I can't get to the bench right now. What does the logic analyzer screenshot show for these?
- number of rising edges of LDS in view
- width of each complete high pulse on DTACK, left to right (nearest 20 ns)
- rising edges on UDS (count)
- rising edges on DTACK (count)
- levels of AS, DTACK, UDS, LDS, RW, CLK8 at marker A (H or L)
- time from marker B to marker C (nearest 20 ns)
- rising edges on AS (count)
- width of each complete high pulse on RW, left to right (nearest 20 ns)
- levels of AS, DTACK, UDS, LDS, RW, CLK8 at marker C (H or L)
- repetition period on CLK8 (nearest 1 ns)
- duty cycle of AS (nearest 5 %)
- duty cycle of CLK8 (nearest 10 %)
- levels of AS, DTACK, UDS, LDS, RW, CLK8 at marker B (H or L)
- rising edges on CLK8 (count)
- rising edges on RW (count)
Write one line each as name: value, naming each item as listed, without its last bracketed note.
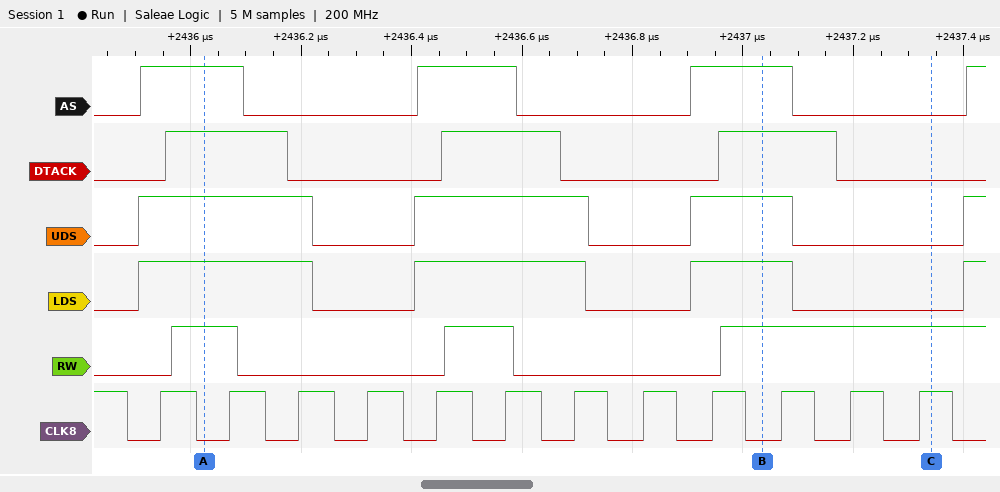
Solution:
number of rising edges of LDS in view: 4
width of each complete high pulse on DTACK, left to right: 220 ns, 220 ns, 220 ns
rising edges on UDS: 4
rising edges on DTACK: 3
levels of AS, DTACK, UDS, LDS, RW, CLK8 at marker A: AS=H, DTACK=H, UDS=H, LDS=H, RW=H, CLK8=L
time from marker B to marker C: 300 ns
rising edges on AS: 4
width of each complete high pulse on RW, left to right: 120 ns, 120 ns
levels of AS, DTACK, UDS, LDS, RW, CLK8 at marker C: AS=L, DTACK=L, UDS=L, LDS=L, RW=H, CLK8=H
repetition period on CLK8: 125 ns
duty cycle of AS: 35 %
duty cycle of CLK8: 50 %
levels of AS, DTACK, UDS, LDS, RW, CLK8 at marker B: AS=H, DTACK=H, UDS=H, LDS=H, RW=H, CLK8=L
rising edges on CLK8: 12
rising edges on RW: 3
